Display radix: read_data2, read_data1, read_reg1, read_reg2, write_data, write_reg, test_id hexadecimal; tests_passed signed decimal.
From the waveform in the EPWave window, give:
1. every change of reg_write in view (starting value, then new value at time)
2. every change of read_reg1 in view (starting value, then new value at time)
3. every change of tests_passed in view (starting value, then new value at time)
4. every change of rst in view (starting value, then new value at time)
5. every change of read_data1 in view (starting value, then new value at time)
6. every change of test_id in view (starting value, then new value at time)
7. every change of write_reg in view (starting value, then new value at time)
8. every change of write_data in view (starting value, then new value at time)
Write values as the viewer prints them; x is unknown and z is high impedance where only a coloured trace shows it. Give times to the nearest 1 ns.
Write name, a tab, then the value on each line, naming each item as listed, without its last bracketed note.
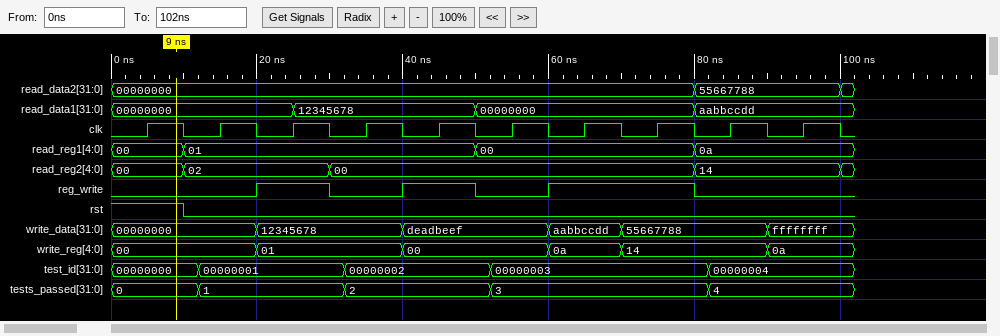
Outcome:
every change of reg_write in view	0, 1 at 20 ns, 0 at 30 ns, 1 at 40 ns, 0 at 50 ns, 1 at 60 ns, 0 at 80 ns
every change of read_reg1 in view	00, 01 at 10 ns, 00 at 50 ns, 0a at 80 ns
every change of tests_passed in view	0, 1 at 12 ns, 2 at 32 ns, 3 at 52 ns, 4 at 82 ns
every change of rst in view	1, 0 at 10 ns
every change of read_data1 in view	00000000, 12345678 at 25 ns, 00000000 at 50 ns, aabbccdd at 80 ns
every change of test_id in view	00000000, 00000001 at 12 ns, 00000002 at 32 ns, 00000003 at 52 ns, 00000004 at 82 ns
every change of write_reg in view	00, 01 at 20 ns, 00 at 40 ns, 0a at 60 ns, 14 at 70 ns, 0a at 90 ns
every change of write_data in view	00000000, 12345678 at 20 ns, deadbeef at 40 ns, aabbccdd at 60 ns, 55667788 at 70 ns, ffffffff at 90 ns
